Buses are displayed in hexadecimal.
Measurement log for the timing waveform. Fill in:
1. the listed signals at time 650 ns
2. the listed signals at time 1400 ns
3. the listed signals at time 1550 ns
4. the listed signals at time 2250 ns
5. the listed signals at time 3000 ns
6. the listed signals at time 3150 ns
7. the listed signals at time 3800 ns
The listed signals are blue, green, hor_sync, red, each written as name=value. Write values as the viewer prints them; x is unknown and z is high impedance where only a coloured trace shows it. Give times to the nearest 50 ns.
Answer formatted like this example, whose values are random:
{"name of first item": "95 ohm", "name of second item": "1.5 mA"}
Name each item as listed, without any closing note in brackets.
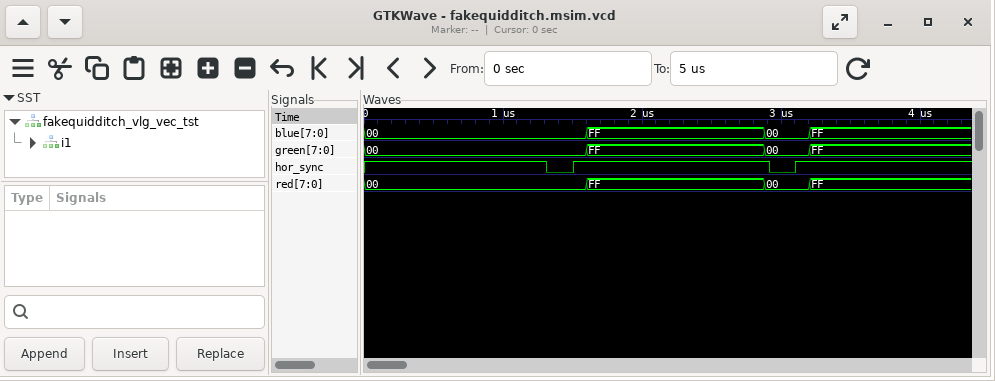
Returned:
{"the listed signals at time 650 ns": "blue=00, green=00, hor_sync=1, red=00", "the listed signals at time 1400 ns": "blue=00, green=00, hor_sync=0, red=00", "the listed signals at time 1550 ns": "blue=00, green=00, hor_sync=1, red=00", "the listed signals at time 2250 ns": "blue=FF, green=FF, hor_sync=1, red=FF", "the listed signals at time 3000 ns": "blue=00, green=00, hor_sync=0, red=00", "the listed signals at time 3150 ns": "blue=00, green=00, hor_sync=1, red=00", "the listed signals at time 3800 ns": "blue=FF, green=FF, hor_sync=1, red=FF"}
